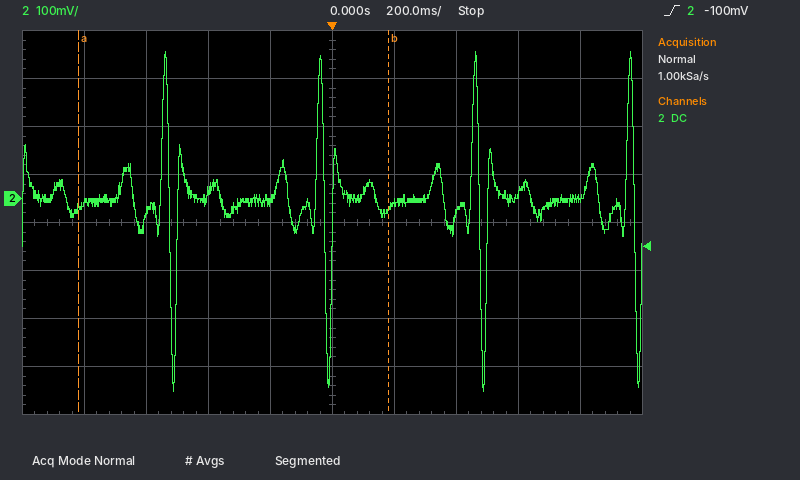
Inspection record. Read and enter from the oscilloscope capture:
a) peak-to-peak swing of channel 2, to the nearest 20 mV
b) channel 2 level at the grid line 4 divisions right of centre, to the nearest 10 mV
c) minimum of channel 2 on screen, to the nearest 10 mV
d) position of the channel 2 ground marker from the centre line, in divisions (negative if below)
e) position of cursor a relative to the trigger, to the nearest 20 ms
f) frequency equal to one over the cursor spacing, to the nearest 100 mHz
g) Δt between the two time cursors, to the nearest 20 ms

700 mV
0 mV
-400 mV
+0.5 div
-820 ms
1.0 Hz
1.00 s
